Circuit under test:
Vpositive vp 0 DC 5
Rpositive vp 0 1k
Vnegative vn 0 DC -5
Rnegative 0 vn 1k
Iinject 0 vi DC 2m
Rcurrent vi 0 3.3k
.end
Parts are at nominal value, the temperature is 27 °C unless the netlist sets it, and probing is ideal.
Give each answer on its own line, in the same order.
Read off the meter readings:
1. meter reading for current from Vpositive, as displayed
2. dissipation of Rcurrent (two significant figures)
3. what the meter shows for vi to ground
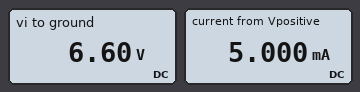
5.000 mA
13 mW
6.60 V
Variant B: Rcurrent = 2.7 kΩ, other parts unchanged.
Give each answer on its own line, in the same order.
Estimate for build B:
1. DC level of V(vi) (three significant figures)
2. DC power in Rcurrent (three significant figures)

5.40 V
10.8 mW
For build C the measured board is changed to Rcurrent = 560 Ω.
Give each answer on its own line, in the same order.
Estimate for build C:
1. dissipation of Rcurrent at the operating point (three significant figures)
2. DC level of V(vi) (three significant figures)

2.24 mW
1.12 V
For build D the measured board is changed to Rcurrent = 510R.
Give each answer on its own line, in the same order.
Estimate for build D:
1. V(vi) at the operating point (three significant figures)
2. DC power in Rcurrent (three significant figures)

1.02 V
2.04 mW
